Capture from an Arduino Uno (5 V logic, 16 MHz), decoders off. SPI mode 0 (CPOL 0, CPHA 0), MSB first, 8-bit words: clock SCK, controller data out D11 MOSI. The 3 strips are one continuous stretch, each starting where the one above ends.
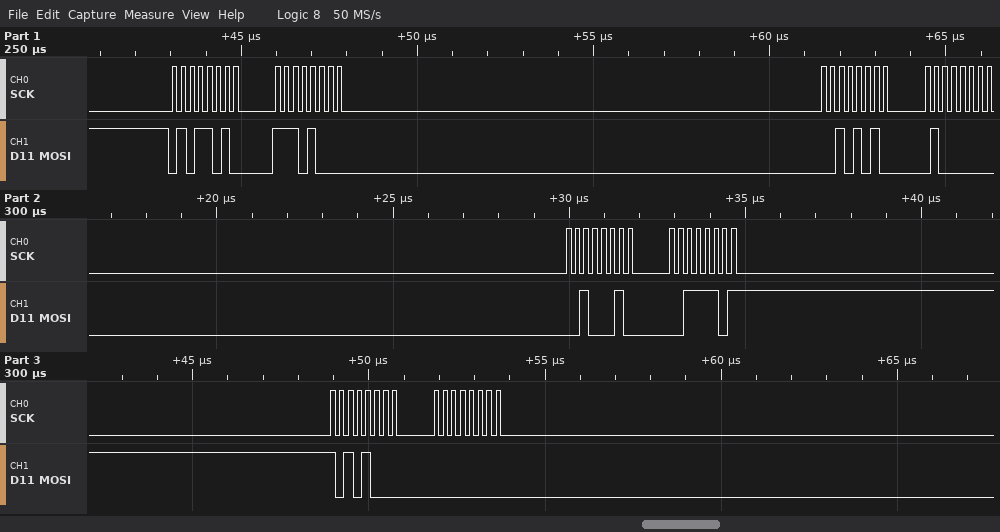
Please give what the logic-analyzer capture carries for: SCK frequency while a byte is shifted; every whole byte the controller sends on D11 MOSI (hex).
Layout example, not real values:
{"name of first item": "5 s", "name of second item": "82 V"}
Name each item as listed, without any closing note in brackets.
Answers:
{"SCK frequency while a byte is shifted": "4 MHz", "every whole byte the controller sends on D11 MOSI": "5A E8 2A 40 22 3D A8 00"}
